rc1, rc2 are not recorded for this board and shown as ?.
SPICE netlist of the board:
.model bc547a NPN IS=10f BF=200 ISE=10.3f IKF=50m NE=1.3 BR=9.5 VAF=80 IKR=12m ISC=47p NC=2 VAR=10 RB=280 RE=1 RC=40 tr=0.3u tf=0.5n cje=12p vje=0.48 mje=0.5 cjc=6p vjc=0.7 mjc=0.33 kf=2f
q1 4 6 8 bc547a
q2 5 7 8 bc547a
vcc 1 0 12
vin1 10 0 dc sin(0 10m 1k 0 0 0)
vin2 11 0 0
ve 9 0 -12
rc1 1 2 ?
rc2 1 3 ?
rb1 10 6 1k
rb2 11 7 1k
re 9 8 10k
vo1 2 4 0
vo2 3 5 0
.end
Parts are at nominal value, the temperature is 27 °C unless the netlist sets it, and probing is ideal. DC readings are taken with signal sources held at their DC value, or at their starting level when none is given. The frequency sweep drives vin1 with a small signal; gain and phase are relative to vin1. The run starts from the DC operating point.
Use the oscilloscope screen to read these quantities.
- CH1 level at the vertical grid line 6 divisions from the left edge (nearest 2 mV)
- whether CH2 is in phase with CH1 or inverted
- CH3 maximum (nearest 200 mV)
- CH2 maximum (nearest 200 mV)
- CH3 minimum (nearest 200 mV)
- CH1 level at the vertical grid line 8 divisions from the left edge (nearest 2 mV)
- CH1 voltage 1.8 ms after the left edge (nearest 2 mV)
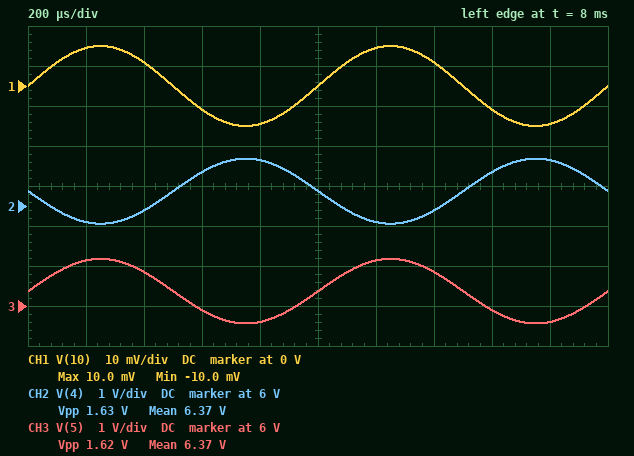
10 mV
inverted
7.2 V
7.2 V
5.6 V
-6 mV
-10 mV
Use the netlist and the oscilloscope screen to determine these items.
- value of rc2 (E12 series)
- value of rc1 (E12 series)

10 kΩ
10 kΩ
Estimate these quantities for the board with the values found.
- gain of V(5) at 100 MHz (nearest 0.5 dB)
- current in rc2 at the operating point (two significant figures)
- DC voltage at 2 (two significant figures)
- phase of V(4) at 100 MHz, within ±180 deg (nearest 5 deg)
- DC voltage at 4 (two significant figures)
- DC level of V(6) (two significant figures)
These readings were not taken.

-10.0 dB
560 µA
6.4 V
10 deg
6.4 V
-4.7 mV
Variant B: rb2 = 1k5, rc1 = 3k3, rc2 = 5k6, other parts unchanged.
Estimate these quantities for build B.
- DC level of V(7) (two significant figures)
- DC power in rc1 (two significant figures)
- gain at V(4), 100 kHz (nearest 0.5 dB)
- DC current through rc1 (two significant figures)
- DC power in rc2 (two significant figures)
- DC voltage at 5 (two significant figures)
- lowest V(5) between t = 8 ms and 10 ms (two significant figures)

-6.6 mV
1.1 mW
28.5 dB
590 µA
1.6 mW
9.0 V
8.5 V
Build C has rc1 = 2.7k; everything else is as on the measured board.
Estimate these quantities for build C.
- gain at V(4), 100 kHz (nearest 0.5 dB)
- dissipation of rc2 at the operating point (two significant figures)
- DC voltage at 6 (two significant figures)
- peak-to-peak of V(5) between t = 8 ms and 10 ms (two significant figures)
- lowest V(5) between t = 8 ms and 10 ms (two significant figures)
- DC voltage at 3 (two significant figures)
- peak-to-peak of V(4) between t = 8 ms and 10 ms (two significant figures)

27.0 dB
3.0 mW
-4.6 mV
1.7 V
5.7 V
6.5 V
450 mV
